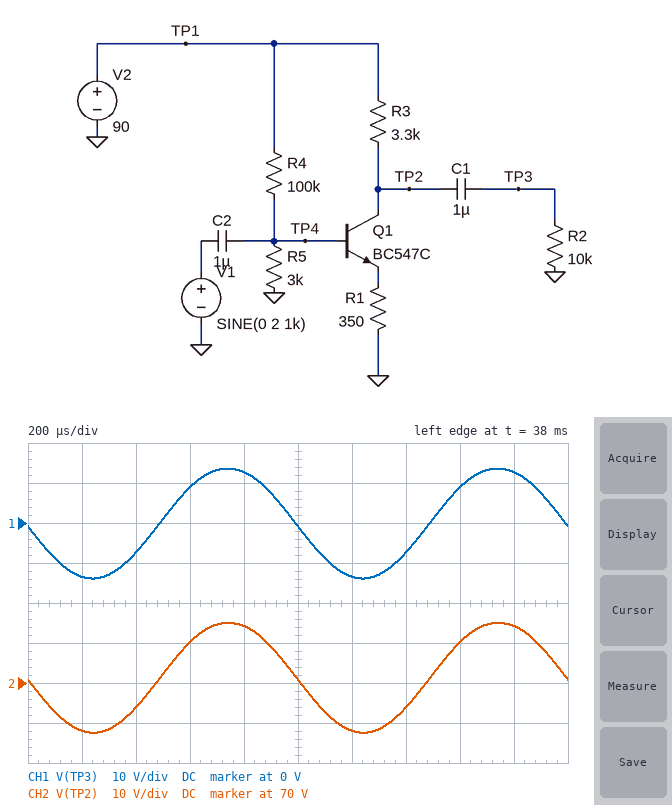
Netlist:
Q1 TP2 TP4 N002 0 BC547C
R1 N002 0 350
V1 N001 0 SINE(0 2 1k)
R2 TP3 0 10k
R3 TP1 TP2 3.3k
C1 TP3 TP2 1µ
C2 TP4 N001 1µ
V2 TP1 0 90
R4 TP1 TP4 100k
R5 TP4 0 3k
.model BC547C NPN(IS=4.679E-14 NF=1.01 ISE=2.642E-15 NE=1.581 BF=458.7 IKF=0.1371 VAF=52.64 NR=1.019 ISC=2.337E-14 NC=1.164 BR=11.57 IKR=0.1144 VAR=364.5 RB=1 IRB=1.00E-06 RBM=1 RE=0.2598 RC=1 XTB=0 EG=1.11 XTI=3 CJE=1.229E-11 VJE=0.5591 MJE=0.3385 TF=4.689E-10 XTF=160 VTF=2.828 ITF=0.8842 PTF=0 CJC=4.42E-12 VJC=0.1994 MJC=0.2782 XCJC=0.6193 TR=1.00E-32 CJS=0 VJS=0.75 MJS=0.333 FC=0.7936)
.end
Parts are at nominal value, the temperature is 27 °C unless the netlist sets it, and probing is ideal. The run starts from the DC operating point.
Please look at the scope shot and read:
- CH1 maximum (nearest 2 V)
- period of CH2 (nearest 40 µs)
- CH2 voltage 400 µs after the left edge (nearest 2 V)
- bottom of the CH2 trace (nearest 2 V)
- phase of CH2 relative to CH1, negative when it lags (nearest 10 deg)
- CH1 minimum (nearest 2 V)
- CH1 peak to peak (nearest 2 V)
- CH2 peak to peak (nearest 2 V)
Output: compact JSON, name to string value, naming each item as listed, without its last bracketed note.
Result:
{"CH1 maximum": "14 V", "period of CH2": "1.00 ms", "CH2 voltage 400 µs after the left edge": "64 V", "bottom of the CH2 trace": "58 V", "phase of CH2 relative to CH1, negative when it lags": "0 deg", "CH1 minimum": "-14 V", "CH1 peak to peak": "28 V", "CH2 peak to peak": "28 V"}
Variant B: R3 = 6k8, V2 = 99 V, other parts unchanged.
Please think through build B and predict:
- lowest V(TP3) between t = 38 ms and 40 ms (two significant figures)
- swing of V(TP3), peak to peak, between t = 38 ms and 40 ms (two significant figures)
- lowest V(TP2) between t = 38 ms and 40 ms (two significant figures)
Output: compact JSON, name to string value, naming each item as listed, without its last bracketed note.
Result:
{"lowest V(TP3) between t = 38 ms and 40 ms": "-23 V", "swing of V(TP3), peak to peak, between t = 38 ms and 40 ms": "45 V", "lowest V(TP2) between t = 38 ms and 40 ms": "33 V"}
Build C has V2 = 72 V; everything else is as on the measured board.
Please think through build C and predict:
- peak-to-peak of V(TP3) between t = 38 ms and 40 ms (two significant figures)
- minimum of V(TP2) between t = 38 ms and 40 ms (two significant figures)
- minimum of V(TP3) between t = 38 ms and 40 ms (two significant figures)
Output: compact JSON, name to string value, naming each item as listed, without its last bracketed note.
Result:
{"peak-to-peak of V(TP3) between t = 38 ms and 40 ms": "24 V", "minimum of V(TP2) between t = 38 ms and 40 ms": "44 V", "minimum of V(TP3) between t = 38 ms and 40 ms": "-13 V"}
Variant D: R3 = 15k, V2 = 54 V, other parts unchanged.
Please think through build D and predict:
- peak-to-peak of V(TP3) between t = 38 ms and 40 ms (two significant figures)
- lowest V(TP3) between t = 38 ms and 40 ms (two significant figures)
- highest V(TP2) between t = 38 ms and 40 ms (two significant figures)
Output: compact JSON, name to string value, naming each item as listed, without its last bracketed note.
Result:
{"peak-to-peak of V(TP3) between t = 38 ms and 40 ms": "32 V", "lowest V(TP3) between t = 38 ms and 40 ms": "-19 V", "highest V(TP2) between t = 38 ms and 40 ms": "34 V"}
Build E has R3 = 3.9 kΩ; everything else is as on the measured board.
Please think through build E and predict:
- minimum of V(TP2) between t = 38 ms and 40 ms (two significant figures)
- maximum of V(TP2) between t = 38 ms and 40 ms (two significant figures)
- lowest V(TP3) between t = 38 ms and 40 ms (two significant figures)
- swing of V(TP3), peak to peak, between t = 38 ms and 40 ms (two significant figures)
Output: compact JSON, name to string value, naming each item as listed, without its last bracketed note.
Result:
{"minimum of V(TP2) between t = 38 ms and 40 ms": "52 V", "maximum of V(TP2) between t = 38 ms and 40 ms": "83 V", "lowest V(TP3) between t = 38 ms and 40 ms": "-16 V", "swing of V(TP3), peak to peak, between t = 38 ms and 40 ms": "31 V"}
